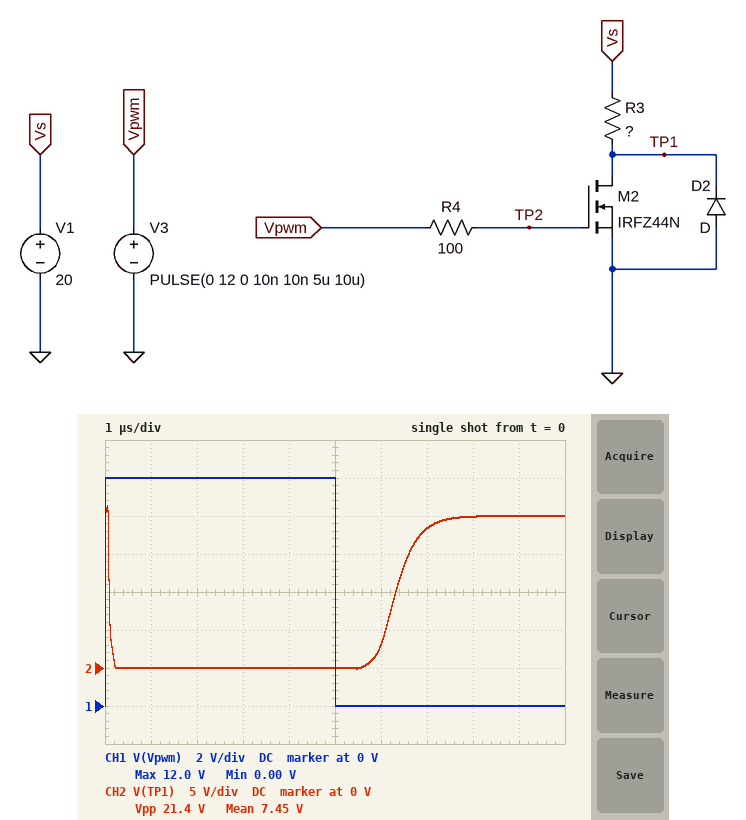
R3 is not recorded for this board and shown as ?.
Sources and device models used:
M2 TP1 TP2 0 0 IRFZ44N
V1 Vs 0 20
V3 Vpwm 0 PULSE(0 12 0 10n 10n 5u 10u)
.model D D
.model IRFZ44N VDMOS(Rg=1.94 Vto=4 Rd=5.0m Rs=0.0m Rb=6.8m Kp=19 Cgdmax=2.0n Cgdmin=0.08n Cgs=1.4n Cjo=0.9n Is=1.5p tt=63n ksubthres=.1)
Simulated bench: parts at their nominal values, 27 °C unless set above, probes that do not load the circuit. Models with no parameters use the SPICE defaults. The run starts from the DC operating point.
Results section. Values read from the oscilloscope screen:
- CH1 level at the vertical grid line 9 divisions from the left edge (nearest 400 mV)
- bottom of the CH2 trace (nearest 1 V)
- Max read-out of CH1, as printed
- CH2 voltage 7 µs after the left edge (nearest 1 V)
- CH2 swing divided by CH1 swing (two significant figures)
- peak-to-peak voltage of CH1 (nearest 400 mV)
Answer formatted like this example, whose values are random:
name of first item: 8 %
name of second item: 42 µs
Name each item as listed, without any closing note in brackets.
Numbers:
CH1 level at the vertical grid line 9 divisions from the left edge: 0 V
bottom of the CH2 trace: 0 V
Max read-out of CH1, as printed: 12.0 V
CH2 voltage 7 µs after the left edge: 18 V
CH2 swing divided by CH1 swing: 1.8
peak-to-peak voltage of CH1: 12.0 V
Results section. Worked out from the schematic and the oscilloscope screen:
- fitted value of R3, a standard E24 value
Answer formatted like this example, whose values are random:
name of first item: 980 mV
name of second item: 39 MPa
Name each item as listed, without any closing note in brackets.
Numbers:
fitted value of R3, a standard E24 value: 1.1 kΩ
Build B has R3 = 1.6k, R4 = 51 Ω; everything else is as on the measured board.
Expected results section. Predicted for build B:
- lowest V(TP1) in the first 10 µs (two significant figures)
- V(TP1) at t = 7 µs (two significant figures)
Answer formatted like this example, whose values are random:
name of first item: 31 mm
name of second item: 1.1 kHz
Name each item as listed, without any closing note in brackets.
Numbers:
lowest V(TP1) in the first 10 µs: -580 mV
V(TP1) at t = 7 µs: 16 V
